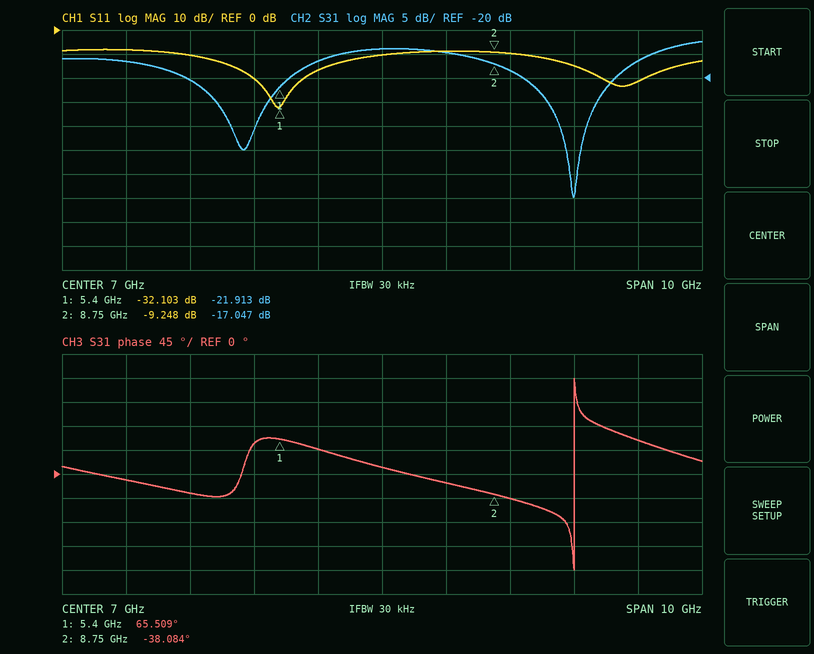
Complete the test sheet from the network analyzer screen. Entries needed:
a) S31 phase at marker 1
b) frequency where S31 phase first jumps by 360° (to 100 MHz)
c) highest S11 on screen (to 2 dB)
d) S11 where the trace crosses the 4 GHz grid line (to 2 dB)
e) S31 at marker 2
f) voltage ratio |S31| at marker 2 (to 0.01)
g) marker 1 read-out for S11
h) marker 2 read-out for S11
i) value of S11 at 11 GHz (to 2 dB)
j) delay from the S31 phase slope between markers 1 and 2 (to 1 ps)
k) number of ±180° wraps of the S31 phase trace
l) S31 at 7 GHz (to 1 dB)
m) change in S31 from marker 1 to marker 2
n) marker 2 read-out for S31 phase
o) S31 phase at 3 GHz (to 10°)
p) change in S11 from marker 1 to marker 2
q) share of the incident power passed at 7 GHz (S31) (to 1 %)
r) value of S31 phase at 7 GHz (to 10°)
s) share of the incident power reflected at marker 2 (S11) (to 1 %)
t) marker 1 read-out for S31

65.509°
10.0 GHz
-8 dB
-10 dB
-17.047 dB
0.14
-32.103 dB
-9.248 dB
-22 dB
86 ps
1
-14 dB
4.866 dB
-38.084°
-10°
22.855 dB
4 %
10°
12 %
-21.913 dB
